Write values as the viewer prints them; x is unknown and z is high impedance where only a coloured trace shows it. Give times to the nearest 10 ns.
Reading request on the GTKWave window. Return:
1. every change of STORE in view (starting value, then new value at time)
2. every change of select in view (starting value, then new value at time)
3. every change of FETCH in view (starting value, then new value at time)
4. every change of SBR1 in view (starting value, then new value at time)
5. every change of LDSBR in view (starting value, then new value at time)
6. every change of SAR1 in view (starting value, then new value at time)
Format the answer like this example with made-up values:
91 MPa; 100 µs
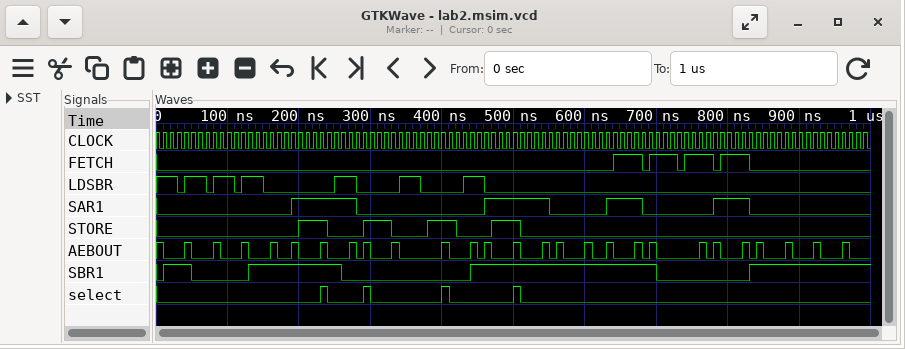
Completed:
0, 1 at 200 ns, 0 at 240 ns, 1 at 290 ns, 0 at 330 ns, 1 at 380 ns, 0 at 420 ns, 1 at 470 ns, 0 at 510 ns; 0, 1 at 230 ns, 0 at 240 ns, 1 at 290 ns, 0 at 300 ns, 1 at 400 ns, 0 at 410 ns, 1 at 500 ns, 0 at 510 ns; 0, 1 at 640 ns, 0 at 680 ns, 1 at 690 ns, 0 at 730 ns, 1 at 740 ns, 0 at 780 ns, 1 at 790 ns, 0 at 830 ns; 0, 1 at 10 ns, 0 at 50 ns, 1 at 130 ns, 0 at 260 ns, 1 at 440 ns, 0 at 700 ns, 1 at 830 ns; 1, 0 at 30 ns, 1 at 40 ns, 0 at 70 ns, 1 at 80 ns, 0 at 110 ns, 1 at 120 ns, 0 at 150 ns, 1 at 250 ns, 0 at 280 ns, 1 at 340 ns, 0 at 370 ns, 1 at 430 ns, 0 at 460 ns; 0, 1 at 190 ns, 0 at 280 ns, 1 at 460 ns, 0 at 550 ns, 1 at 630 ns, 0 at 680 ns, 1 at 780 ns, 0 at 830 ns
